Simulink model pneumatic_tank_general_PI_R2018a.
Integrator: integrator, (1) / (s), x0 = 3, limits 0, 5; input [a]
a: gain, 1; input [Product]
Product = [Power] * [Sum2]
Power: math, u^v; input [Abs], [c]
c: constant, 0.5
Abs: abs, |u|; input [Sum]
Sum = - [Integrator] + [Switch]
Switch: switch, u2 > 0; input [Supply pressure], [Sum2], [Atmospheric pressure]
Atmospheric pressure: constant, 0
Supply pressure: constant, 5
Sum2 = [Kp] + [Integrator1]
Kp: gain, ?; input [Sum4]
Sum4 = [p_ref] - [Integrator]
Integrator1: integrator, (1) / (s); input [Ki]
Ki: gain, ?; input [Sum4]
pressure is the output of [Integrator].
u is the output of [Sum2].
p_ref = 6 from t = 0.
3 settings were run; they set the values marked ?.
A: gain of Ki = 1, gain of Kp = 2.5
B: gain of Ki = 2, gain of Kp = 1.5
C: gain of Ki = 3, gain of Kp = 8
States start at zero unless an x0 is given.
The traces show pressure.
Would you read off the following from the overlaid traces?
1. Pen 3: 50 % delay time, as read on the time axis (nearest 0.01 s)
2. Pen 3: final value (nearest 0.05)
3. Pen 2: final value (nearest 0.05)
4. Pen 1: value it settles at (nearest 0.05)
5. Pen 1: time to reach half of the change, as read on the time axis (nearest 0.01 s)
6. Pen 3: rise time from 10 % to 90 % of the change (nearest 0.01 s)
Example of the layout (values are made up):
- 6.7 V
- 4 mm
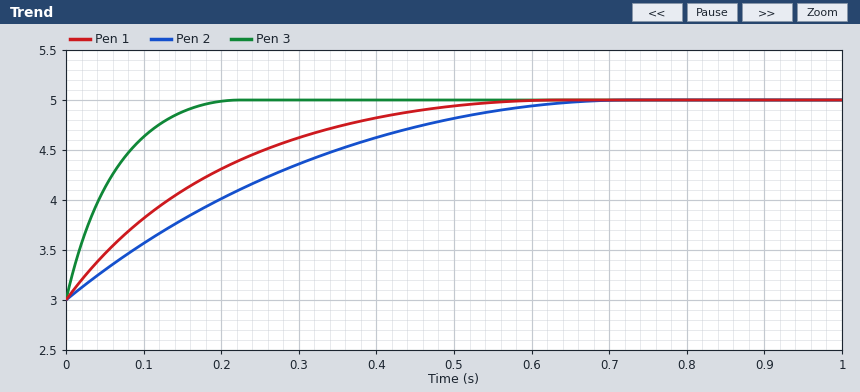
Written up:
- 0.04 s
- 5.00
- 5.00
- 5.00
- 0.13 s
- 0.12 s
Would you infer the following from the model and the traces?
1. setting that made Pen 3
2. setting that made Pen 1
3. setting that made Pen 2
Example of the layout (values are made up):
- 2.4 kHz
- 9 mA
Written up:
- C
- A
- B
